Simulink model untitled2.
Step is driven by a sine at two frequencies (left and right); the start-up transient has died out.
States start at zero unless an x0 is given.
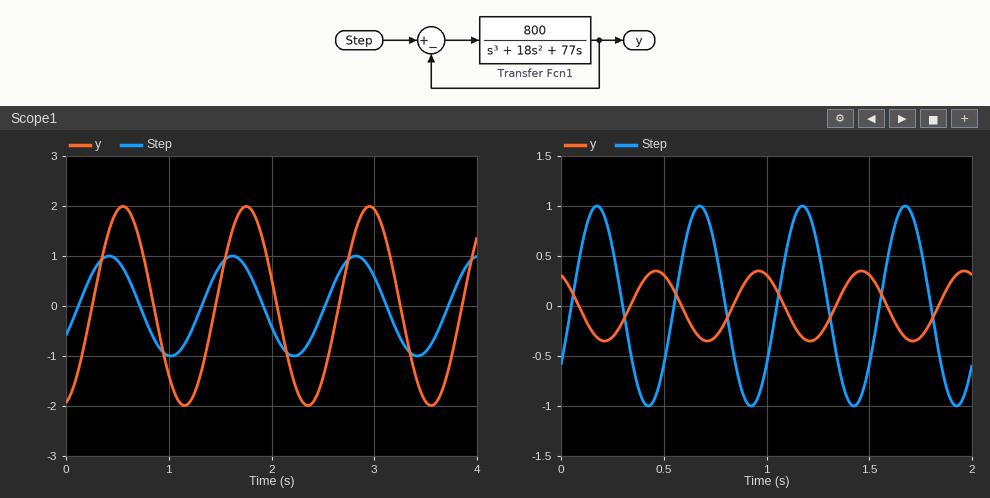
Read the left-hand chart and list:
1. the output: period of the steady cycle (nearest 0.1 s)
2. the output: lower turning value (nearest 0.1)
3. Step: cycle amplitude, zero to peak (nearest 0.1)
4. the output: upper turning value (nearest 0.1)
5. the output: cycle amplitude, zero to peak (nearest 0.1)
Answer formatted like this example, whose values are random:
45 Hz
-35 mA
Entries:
1.2 s
-2.0
1.0
2.0
2.0
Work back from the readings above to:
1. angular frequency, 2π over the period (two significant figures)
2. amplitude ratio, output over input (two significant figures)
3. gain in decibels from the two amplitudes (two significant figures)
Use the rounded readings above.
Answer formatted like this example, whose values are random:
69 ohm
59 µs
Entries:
5.2 rad/s
2.0
6.0 dB
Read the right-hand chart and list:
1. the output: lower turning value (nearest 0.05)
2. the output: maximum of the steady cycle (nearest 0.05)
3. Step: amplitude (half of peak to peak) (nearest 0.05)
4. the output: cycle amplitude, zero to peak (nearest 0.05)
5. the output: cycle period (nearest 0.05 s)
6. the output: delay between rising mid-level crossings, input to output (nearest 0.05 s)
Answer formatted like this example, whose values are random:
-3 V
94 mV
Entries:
-0.35
0.35
1.00
0.35
0.50 s
0.30 s
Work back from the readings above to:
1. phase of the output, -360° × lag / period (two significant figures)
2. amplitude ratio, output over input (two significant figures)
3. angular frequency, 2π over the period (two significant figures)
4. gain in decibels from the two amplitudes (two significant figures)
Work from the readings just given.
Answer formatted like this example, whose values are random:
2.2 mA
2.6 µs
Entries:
-220°
0.35
13 rad/s
-9.1 dB
